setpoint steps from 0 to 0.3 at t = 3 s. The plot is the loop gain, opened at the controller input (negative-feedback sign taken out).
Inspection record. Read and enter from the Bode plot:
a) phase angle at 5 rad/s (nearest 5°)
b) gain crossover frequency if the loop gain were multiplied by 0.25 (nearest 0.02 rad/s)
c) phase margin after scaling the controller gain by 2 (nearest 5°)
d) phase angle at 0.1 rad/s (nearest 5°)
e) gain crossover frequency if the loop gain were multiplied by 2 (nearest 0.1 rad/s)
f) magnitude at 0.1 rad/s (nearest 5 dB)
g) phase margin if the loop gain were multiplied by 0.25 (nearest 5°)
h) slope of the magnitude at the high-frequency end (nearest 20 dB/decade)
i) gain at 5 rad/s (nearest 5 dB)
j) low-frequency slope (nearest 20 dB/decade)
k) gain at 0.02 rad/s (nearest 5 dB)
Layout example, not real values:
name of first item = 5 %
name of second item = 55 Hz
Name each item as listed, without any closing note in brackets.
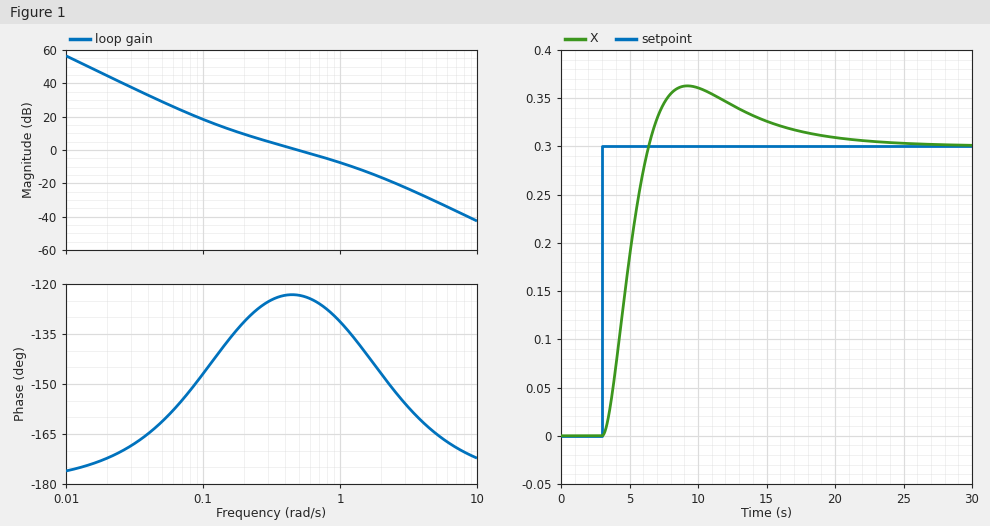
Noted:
phase angle at 5 rad/s = -165°
gain crossover frequency if the loop gain were multiplied by 0.25 = 0.16 rad/s
phase margin after scaling the controller gain by 2 = 50°
phase angle at 0.1 rad/s = -145°
gain crossover frequency if the loop gain were multiplied by 2 = 0.9 rad/s
magnitude at 0.1 rad/s = 20 dB
phase margin if the loop gain were multiplied by 0.25 = 45°
slope of the magnitude at the high-frequency end = -40 dB/decade
gain at 5 rad/s = -30 dB
low-frequency slope = -40 dB/decade
gain at 0.02 rad/s = 45 dB
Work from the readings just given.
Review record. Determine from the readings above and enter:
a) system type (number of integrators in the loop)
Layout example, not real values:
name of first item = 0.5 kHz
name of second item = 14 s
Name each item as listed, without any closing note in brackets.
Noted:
system type = 2
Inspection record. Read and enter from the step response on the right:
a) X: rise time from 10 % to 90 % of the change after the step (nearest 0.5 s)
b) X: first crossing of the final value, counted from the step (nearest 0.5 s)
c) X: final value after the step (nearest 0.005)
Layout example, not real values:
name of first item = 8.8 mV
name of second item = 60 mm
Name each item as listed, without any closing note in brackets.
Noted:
X: rise time from 10 % to 90 % of the change after the step = 2.5 s
X: first crossing of the final value, counted from the step = 3.5 s
X: final value after the step = 0.300
